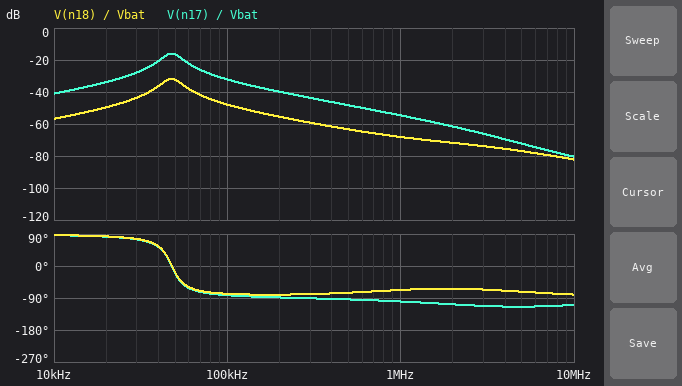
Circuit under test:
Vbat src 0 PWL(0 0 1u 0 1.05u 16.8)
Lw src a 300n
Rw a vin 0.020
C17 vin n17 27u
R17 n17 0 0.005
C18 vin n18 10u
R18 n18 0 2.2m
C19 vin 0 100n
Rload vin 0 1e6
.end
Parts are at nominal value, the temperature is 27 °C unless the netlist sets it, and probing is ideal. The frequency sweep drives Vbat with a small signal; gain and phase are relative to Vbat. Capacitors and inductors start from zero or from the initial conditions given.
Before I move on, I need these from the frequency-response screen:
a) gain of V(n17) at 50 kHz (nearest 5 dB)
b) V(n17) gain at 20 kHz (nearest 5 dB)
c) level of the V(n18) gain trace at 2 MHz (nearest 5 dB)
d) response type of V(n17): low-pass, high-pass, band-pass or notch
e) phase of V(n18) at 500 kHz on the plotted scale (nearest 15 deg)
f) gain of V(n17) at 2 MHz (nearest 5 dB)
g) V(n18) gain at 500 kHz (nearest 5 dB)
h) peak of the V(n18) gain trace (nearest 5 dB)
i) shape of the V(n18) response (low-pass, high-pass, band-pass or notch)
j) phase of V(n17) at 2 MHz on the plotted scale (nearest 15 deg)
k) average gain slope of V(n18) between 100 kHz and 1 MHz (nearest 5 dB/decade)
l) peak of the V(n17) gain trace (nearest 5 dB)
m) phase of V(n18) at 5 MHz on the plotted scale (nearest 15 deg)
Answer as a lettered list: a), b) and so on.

a) -15 dB
b) -35 dB
c) -70 dB
d) band-pass
e) -75 deg
f) -60 dB
g) -65 dB
h) -30 dB
i) band-pass
j) -105 deg
k) -20 dB/decade
l) -15 dB
m) -75 deg
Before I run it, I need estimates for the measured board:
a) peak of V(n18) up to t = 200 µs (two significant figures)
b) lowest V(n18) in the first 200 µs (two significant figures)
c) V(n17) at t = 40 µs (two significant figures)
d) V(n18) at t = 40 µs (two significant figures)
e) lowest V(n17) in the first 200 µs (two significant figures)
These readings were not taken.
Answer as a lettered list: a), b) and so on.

a) 92 mV
b) -62 mV
c) -130 mV
d) -21 mV
e) -380 mV
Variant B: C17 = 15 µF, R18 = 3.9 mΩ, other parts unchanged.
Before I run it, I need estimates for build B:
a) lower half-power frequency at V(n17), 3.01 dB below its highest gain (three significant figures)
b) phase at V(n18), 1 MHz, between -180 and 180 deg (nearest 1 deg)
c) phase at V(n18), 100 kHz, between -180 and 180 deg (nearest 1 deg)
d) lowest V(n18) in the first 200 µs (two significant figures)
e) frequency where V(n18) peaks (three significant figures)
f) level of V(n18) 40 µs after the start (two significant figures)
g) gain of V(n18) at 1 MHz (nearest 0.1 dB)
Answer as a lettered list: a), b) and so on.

a) 52.4 kHz
b) -83 deg
c) -79 deg
d) -150 mV
e) 58.0 kHz
f) 56 mV
g) -61.2 dB
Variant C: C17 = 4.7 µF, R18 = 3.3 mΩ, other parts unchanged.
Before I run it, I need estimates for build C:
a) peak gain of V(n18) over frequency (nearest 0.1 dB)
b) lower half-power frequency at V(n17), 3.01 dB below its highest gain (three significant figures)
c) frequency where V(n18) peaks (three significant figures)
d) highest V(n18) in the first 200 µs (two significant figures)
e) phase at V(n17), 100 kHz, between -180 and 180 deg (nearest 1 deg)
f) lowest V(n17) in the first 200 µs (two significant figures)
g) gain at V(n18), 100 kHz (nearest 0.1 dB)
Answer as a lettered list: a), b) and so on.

a) -19.9 dB
b) 69.9 kHz
c) 75.5 kHz
d) 230 mV
e) -75 deg
f) -130 mV
g) -31.5 dB
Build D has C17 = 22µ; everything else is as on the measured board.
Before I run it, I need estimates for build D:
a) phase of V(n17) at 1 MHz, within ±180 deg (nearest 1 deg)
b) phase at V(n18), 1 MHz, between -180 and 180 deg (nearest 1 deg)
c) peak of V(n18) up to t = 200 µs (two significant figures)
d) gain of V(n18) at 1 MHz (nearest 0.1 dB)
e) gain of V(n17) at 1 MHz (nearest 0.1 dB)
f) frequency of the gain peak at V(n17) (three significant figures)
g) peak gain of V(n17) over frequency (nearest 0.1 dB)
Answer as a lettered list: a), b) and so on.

a) -99 deg
b) -72 deg
c) 100 mV
d) -67.5 dB
e) -55.1 dB
f) 51.3 kHz
g) -16.4 dB
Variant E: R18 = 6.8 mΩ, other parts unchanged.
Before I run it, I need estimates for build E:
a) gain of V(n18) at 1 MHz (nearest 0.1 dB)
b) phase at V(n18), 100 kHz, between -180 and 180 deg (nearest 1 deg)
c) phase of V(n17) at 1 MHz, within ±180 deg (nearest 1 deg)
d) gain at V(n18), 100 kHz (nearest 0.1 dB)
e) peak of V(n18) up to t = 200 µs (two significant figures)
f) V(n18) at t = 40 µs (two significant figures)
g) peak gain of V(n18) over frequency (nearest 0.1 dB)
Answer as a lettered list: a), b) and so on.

a) -59.0 dB
b) -79 deg
c) -95 deg
d) -38.1 dB
e) 280 mV
f) -63 mV
g) -22.0 dB
